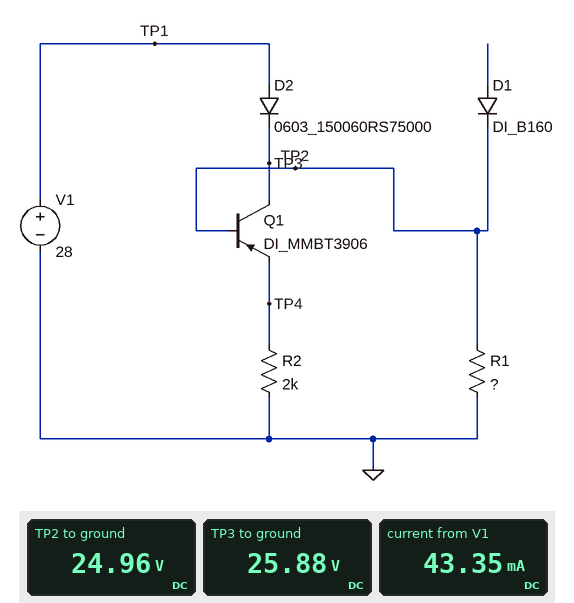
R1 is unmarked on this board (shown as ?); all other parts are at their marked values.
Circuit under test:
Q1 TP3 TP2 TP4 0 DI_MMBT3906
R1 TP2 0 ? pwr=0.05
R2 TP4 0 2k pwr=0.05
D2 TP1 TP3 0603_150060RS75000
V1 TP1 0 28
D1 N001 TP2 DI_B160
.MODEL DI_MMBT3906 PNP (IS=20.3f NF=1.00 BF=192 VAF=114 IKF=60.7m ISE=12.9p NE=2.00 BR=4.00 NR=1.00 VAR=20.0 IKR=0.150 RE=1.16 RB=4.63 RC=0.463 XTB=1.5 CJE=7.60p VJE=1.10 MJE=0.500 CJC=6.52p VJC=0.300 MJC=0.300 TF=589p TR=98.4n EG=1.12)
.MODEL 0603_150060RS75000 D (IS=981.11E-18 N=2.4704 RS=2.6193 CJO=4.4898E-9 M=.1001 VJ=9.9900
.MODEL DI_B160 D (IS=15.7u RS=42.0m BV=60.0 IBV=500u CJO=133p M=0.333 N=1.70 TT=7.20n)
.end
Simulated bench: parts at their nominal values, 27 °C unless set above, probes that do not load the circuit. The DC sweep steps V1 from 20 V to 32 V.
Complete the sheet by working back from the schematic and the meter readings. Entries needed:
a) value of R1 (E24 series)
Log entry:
820 Ω
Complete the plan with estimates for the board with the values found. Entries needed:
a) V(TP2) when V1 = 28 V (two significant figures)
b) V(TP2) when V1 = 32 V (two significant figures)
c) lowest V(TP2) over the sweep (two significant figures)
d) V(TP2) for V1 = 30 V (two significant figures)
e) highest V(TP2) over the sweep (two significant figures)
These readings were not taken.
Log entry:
25 V
29 V
17 V
27 V
29 V
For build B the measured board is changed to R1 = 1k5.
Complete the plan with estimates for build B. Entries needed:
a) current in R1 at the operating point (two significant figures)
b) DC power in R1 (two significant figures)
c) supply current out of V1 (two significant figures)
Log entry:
17 mA
420 mW
30 mA
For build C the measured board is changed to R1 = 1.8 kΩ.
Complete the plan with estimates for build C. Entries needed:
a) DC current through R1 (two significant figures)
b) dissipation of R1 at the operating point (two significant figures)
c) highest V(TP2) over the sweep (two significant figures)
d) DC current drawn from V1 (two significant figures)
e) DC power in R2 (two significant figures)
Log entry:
14 mA
350 mW
29 V
27 mA
340 mW
